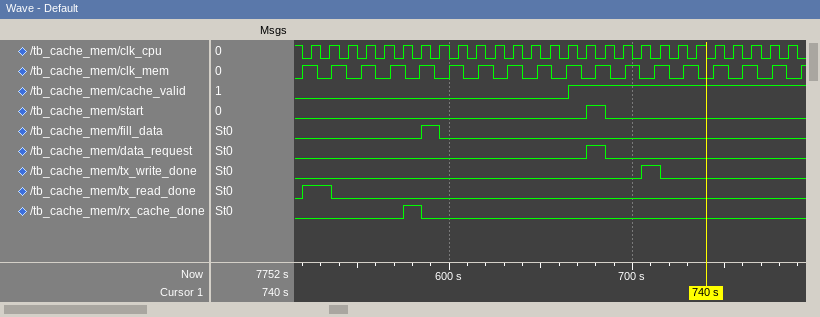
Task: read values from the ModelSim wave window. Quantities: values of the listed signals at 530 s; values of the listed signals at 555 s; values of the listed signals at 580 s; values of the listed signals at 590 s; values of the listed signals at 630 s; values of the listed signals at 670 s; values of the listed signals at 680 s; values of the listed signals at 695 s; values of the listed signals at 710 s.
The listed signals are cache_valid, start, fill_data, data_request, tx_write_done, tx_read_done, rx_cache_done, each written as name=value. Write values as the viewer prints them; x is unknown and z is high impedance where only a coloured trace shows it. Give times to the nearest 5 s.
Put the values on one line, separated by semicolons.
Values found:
cache_valid=0, start=0, fill_data=0, data_request=0, tx_write_done=0, tx_read_done=1, rx_cache_done=0; cache_valid=0, start=0, fill_data=0, data_request=0, tx_write_done=0, tx_read_done=0, rx_cache_done=0; cache_valid=0, start=0, fill_data=0, data_request=0, tx_write_done=0, tx_read_done=0, rx_cache_done=1; cache_valid=0, start=0, fill_data=1, data_request=0, tx_write_done=0, tx_read_done=0, rx_cache_done=0; cache_valid=0, start=0, fill_data=0, data_request=0, tx_write_done=0, tx_read_done=0, rx_cache_done=0; cache_valid=1, start=0, fill_data=0, data_request=0, tx_write_done=0, tx_read_done=0, rx_cache_done=0; cache_valid=1, start=1, fill_data=0, data_request=1, tx_write_done=0, tx_read_done=0, rx_cache_done=0; cache_valid=1, start=0, fill_data=0, data_request=0, tx_write_done=0, tx_read_done=0, rx_cache_done=0; cache_valid=1, start=0, fill_data=0, data_request=0, tx_write_done=1, tx_read_done=0, rx_cache_done=0
